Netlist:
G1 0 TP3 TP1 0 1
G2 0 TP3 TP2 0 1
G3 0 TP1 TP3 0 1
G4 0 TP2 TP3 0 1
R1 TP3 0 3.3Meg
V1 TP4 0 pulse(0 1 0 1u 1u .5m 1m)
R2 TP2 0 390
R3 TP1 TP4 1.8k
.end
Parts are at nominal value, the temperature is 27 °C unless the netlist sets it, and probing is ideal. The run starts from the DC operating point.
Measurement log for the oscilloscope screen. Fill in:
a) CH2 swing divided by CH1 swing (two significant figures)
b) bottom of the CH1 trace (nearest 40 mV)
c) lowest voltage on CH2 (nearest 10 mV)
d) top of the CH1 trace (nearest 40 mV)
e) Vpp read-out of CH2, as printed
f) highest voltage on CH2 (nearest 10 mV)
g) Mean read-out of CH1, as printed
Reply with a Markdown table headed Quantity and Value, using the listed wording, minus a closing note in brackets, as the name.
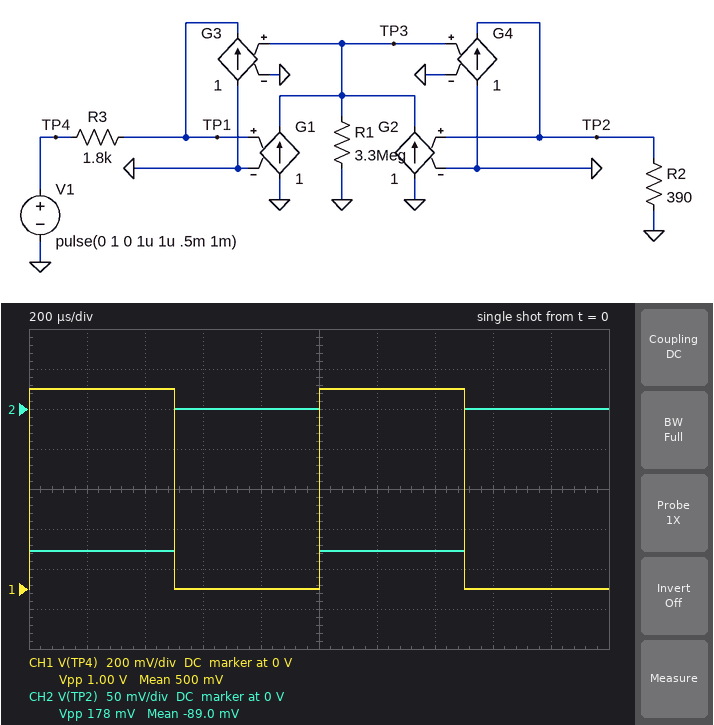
| Quantity | Value |
|---|---|
| CH2 swing divided by CH1 swing | 0.18 |
| bottom of the CH1 trace | 0 V |
| lowest voltage on CH2 | -180 mV |
| top of the CH1 trace | 1.00 V |
| Vpp read-out of CH2, as printed | 178 mV |
| highest voltage on CH2 | 0 V |
| Mean read-out of CH1, as printed | 500 mV |
